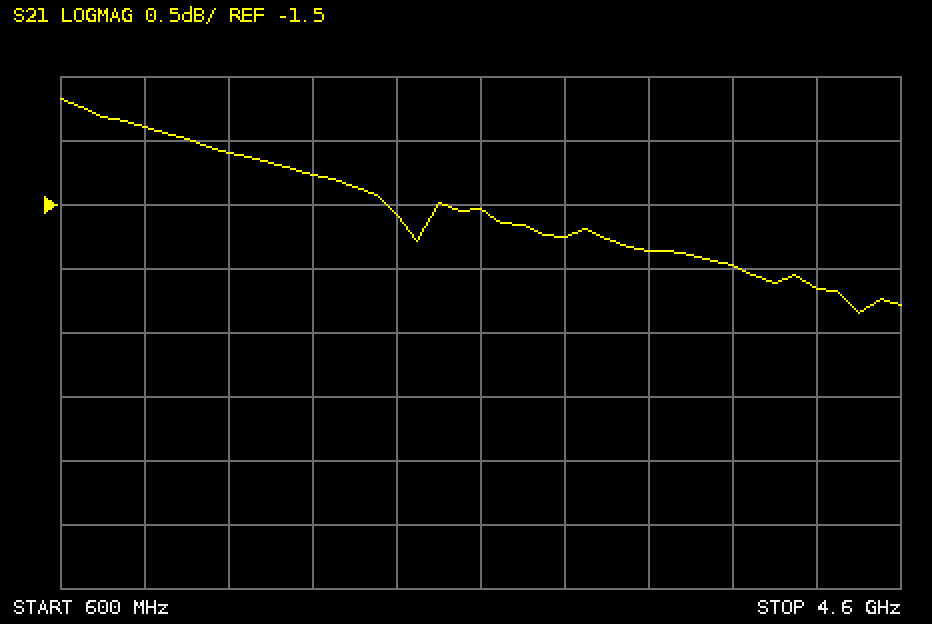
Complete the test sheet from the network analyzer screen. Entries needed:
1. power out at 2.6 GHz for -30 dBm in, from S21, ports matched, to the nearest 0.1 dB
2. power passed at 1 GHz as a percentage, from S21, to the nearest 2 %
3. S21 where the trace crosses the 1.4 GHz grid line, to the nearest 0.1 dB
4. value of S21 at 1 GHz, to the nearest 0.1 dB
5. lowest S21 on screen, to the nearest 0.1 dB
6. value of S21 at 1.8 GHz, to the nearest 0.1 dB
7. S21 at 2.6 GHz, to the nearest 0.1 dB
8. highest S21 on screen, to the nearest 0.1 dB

-31.5 dBm
82 %
-1.1 dB
-0.9 dB
-2.3 dB
-1.3 dB
-1.5 dB
-0.7 dB
